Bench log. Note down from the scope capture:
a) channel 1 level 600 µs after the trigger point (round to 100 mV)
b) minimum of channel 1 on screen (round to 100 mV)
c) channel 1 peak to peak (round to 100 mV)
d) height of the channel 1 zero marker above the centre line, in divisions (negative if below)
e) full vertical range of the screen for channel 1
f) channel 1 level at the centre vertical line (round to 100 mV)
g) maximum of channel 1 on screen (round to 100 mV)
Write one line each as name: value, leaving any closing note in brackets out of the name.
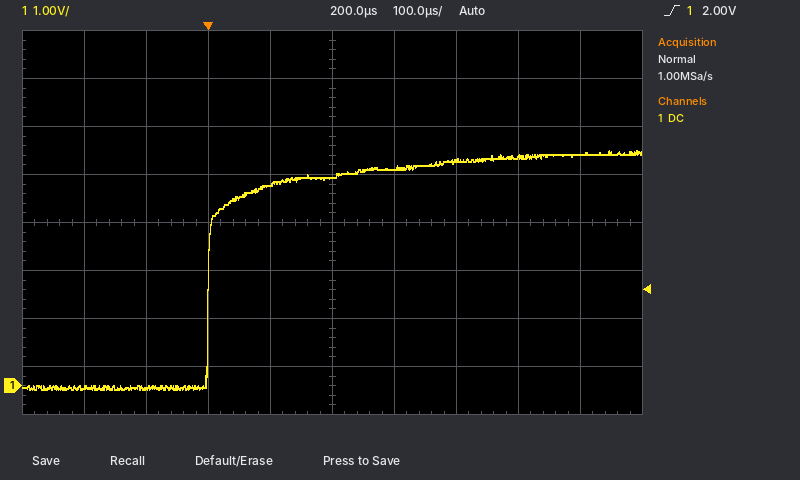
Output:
channel 1 level 600 µs after the trigger point: 4.8 V
minimum of channel 1 on screen: -100 mV
channel 1 peak to peak: 5.0 V
height of the channel 1 zero marker above the centre line, in divisions: -3.4 div
full vertical range of the screen for channel 1: 8 V
channel 1 level at the centre vertical line: 4.3 V
maximum of channel 1 on screen: 4.9 V
